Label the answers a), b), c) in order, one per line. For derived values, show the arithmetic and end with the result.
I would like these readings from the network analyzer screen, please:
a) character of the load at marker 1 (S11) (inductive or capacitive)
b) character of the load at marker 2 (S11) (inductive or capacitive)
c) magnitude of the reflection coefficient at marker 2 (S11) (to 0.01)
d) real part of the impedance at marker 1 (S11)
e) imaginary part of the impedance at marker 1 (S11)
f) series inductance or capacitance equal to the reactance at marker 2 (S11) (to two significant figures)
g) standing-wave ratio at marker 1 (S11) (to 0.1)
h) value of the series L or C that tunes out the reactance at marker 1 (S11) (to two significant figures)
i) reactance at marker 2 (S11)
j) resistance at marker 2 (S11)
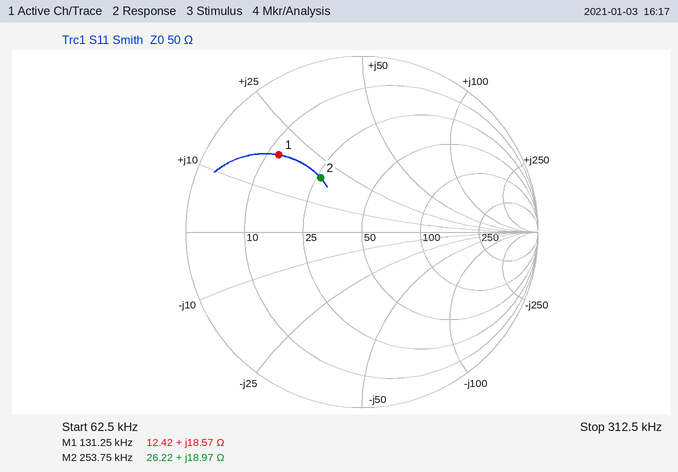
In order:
a) inductive
b) inductive
c) 0.39
d) 12.42 Ω
e) +18.57 Ω
f) L = 18.97 Ω/(2π × 253.75 kHz) ≈ 12 µH
g) 4.6
h) C = 1/(2π × 131.25 kHz × 18.57 Ω) ≈ 65 nF
i) +18.97 Ω
j) 26.22 Ω
